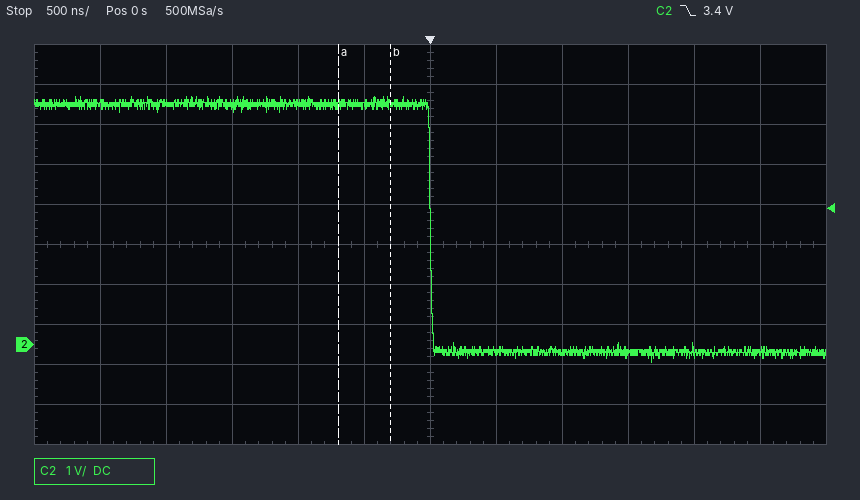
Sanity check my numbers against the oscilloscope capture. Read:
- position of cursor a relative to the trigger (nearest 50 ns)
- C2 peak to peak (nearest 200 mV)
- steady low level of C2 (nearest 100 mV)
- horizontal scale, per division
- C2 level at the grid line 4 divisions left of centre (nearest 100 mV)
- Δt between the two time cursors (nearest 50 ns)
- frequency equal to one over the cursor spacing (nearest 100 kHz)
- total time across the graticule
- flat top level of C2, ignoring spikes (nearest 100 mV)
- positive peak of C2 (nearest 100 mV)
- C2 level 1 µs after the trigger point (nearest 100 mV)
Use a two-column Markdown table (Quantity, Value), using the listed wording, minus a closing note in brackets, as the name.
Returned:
| Quantity | Value |
|---|---|
| position of cursor a relative to the trigger | -700 ns |
| C2 peak to peak | 6.6 V |
| steady low level of C2 | -200 mV |
| horizontal scale, per division | 500 ns |
| C2 level at the grid line 4 divisions left of centre | 6.0 V |
| Δt between the two time cursors | 400 ns |
| frequency equal to one over the cursor spacing | 2.5 MHz |
| total time across the graticule | 6 µs |
| flat top level of C2, ignoring spikes | 6.0 V |
| positive peak of C2 | 6.2 V |
| C2 level 1 µs after the trigger point | -200 mV |
